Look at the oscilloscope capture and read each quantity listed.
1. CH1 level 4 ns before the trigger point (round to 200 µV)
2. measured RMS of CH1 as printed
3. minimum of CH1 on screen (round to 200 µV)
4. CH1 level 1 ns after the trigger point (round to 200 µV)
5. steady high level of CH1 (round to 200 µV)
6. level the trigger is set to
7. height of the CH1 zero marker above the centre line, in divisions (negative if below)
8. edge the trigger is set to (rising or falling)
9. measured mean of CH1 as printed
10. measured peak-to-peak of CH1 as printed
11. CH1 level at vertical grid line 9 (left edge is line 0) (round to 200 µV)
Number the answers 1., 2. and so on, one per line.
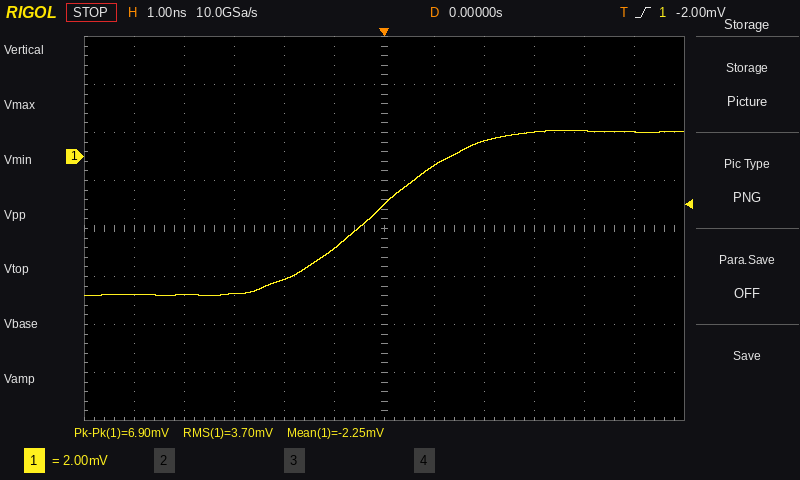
1. -5.8 mV
2. 3.70 mV
3. -5.8 mV
4. -400 µV
5. 1.0 mV
6. -2.00 mV
7. +1.5 div
8. rising
9. -2.25 mV
10. 6.90 mV
11. 1.0 mV
